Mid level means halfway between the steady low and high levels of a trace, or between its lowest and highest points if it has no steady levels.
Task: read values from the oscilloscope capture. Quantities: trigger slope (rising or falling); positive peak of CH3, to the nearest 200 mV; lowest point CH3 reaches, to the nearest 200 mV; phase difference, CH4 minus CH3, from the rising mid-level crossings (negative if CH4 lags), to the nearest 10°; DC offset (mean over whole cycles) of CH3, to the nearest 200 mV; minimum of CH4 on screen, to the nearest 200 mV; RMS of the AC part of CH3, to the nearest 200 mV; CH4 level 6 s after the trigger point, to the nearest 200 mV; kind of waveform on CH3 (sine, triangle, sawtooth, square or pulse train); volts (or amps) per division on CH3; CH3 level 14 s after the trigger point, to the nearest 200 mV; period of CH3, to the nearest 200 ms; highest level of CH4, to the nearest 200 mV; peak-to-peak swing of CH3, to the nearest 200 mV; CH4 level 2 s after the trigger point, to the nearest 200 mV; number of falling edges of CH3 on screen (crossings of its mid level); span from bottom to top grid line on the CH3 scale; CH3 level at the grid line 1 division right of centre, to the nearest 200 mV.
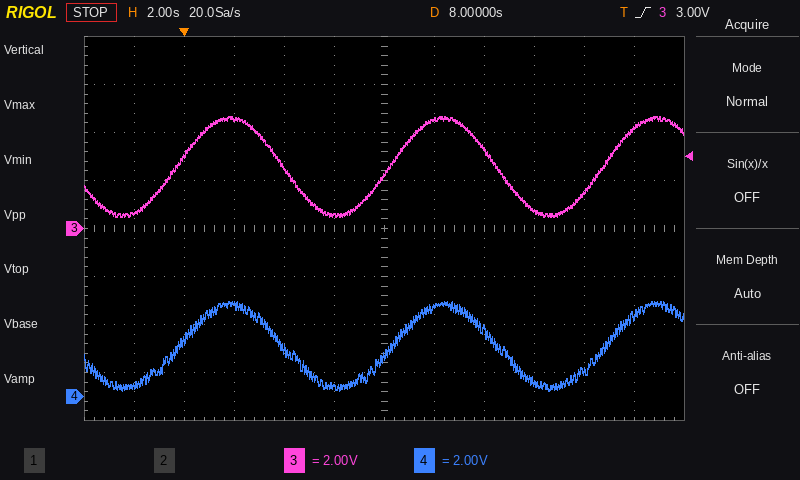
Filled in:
rising
4.6 V
400 mV
0°
2.6 V
200 mV
1.4 V
400 mV
sine
2 V
800 mV
8.6 s
4.0 V
4.2 V
3.8 V
2
16 V
4.6 V
